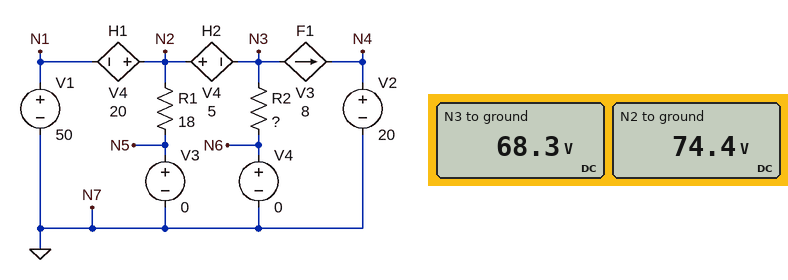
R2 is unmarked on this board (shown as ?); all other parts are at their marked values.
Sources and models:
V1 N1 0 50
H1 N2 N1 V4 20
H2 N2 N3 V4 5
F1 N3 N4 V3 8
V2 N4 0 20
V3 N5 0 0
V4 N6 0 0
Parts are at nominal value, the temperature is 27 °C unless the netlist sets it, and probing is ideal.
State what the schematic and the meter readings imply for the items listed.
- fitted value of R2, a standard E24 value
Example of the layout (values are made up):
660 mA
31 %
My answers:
56 Ω
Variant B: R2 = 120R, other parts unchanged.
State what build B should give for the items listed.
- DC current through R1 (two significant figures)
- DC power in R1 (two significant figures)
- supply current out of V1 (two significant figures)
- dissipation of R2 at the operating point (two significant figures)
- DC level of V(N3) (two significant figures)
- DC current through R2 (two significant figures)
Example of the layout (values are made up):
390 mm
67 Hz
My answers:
3.3 A
200 W
30 A
27 W
57 V
480 mA
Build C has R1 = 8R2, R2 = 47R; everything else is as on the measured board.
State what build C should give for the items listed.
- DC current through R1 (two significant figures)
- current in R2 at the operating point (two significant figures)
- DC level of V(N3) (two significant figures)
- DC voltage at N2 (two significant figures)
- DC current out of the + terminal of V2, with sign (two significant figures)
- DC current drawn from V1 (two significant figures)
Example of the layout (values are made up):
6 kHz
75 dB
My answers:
9.9 A
1.6 A
73 V
81 V
-79 A
91 A
